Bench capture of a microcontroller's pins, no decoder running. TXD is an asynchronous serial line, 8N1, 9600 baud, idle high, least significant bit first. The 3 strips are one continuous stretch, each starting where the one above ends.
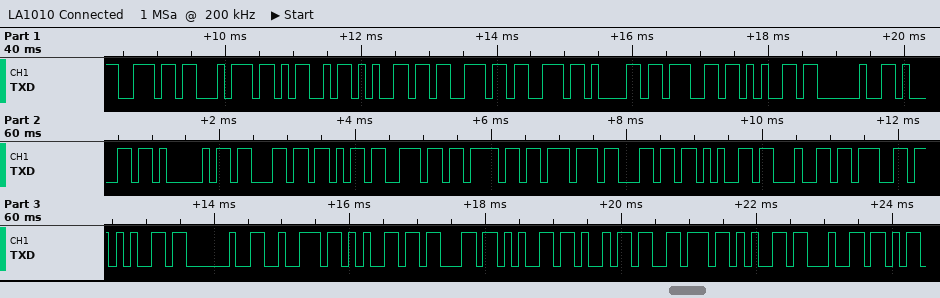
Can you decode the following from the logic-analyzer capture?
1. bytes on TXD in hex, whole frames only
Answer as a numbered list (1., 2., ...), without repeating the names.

1. 6E 74 4D 65 73 73 61 67 65 20 61 41 63 6B 6E 6F 77 6C 65 64 67 65 20 72 65 63 65 69 76 65 64
